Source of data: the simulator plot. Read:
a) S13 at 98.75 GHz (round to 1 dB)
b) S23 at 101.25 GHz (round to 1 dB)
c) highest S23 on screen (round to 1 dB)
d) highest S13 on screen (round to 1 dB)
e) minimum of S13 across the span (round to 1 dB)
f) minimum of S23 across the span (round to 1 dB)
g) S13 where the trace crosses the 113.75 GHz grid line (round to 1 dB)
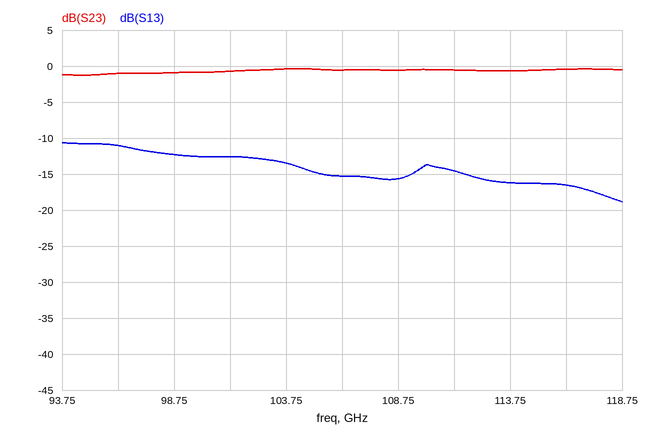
-12 dB
-1 dB
0 dB
-11 dB
-19 dB
-1 dB
-16 dB
